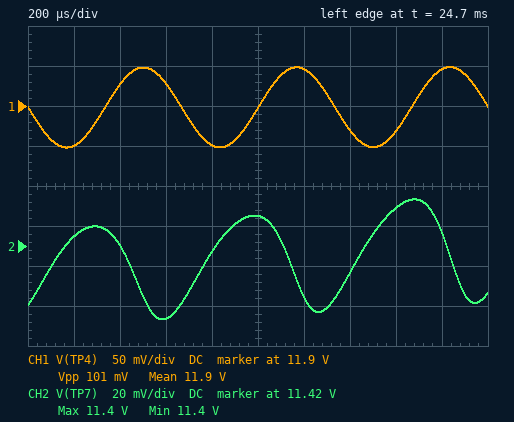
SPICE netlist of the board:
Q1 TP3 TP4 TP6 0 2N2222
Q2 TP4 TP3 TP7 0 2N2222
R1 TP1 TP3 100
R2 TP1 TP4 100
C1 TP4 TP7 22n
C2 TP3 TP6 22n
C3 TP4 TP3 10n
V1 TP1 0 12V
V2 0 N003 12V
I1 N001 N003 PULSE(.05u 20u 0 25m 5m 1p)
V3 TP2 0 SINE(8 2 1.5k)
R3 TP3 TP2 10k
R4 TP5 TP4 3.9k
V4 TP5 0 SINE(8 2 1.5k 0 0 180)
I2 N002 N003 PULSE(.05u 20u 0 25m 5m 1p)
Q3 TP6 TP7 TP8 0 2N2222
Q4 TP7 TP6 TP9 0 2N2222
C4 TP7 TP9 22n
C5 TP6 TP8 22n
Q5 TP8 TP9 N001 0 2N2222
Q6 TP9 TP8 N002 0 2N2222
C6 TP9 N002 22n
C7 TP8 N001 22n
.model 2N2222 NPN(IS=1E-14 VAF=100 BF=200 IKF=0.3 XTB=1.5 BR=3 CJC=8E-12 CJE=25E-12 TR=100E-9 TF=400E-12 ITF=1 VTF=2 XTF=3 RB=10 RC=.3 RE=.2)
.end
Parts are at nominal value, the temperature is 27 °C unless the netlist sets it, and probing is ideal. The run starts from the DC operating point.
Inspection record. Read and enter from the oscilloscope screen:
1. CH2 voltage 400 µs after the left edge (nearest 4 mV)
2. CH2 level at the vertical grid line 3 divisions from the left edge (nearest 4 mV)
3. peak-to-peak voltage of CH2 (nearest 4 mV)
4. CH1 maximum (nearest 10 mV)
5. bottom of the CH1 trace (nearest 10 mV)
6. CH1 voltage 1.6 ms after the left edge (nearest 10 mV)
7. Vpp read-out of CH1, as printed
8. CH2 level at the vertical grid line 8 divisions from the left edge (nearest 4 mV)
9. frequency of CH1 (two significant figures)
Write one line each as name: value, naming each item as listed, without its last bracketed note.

CH2 voltage 400 µs after the left edge: 11.420 V
CH2 level at the vertical grid line 3 divisions from the left edge: 11.384 V
peak-to-peak voltage of CH2: 60 mV
CH1 maximum: 11.95 V
bottom of the CH1 trace: 11.85 V
CH1 voltage 1.6 ms after the left edge: 11.87 V
Vpp read-out of CH1, as printed: 101 mV
CH2 level at the vertical grid line 8 divisions from the left edge: 11.440 V
frequency of CH1: 1.5 kHz
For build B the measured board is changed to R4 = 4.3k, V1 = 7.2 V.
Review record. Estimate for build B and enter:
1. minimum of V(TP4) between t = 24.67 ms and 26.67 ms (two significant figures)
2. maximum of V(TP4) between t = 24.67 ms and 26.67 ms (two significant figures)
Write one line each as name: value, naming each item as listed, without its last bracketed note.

minimum of V(TP4) between t = 24.67 ms and 26.67 ms: 7.2 V
maximum of V(TP4) between t = 24.67 ms and 26.67 ms: 7.3 V
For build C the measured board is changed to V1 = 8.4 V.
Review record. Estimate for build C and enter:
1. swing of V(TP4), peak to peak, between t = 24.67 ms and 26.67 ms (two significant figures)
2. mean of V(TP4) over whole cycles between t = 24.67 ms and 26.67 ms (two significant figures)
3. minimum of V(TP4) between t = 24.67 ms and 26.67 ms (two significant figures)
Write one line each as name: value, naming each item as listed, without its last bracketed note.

swing of V(TP4), peak to peak, between t = 24.67 ms and 26.67 ms: 100 mV
mean of V(TP4) over whole cycles between t = 24.67 ms and 26.67 ms: 8.4 V
minimum of V(TP4) between t = 24.67 ms and 26.67 ms: 8.3 V
